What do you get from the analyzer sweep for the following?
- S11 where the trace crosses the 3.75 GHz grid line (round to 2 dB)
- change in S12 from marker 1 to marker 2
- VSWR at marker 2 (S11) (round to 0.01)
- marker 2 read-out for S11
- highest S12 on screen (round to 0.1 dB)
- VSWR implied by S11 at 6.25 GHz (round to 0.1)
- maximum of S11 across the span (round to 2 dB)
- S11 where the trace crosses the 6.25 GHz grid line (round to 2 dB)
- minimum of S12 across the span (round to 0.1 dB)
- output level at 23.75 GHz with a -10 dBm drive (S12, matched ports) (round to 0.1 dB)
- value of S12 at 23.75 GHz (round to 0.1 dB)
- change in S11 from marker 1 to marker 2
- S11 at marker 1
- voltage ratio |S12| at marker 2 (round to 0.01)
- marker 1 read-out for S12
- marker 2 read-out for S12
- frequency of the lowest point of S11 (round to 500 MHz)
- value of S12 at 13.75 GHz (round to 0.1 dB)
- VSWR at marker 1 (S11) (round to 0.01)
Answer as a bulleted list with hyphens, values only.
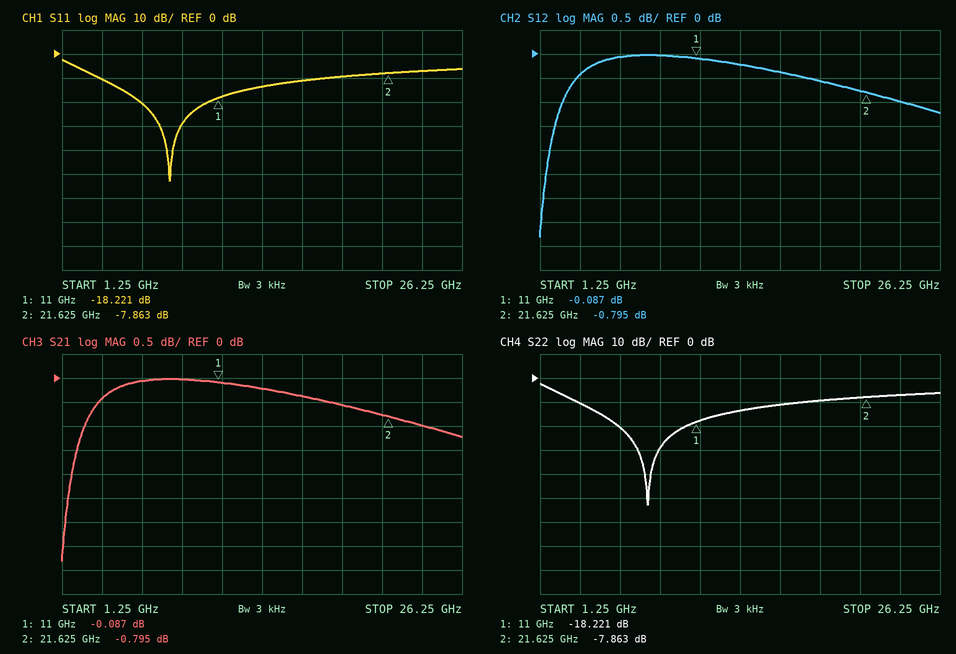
- -10 dB
- -0.708 dB
- 2.36
- -7.863 dB
- 0.0 dB
- 1.2
- -2 dB
- -20 dB
- -3.8 dB
- -11.0 dBm
- -1.0 dB
- 10.358 dB
- -18.221 dB
- 0.91
- -0.087 dB
- -0.795 dB
- 8.0 GHz
- -0.2 dB
- 1.28
